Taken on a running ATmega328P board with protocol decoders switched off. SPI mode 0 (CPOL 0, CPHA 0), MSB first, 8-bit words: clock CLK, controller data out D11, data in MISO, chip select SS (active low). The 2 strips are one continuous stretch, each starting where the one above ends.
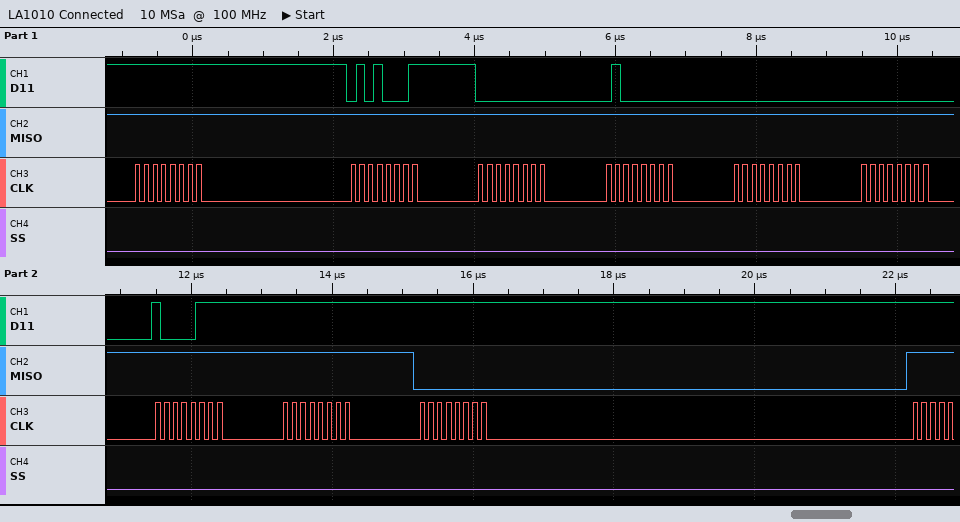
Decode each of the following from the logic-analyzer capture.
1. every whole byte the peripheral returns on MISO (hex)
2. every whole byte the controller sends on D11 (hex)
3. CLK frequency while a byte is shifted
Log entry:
FF FF FF FF FF FF FF FF 00
FF 51 00 40 00 00 87 FF FF
8 MHz
